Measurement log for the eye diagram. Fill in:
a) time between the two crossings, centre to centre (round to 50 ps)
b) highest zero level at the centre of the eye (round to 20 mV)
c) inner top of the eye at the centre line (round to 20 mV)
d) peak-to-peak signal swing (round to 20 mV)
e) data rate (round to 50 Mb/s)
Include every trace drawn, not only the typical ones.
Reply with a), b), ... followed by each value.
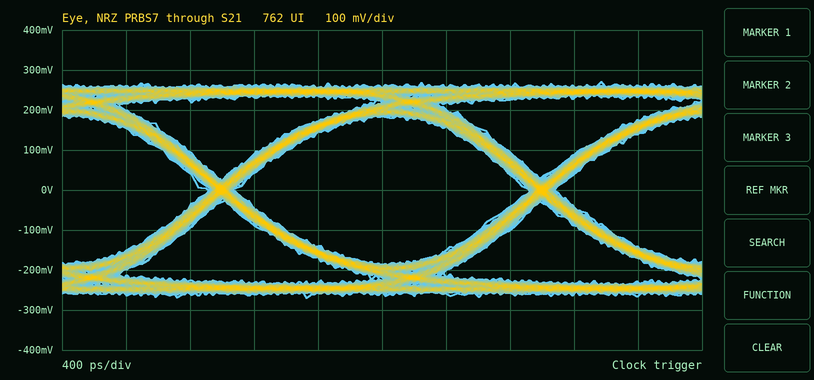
a) 2.00 ns
b) -180 mV
c) 180 mV
d) 540 mV
e) 500 Mb/s
